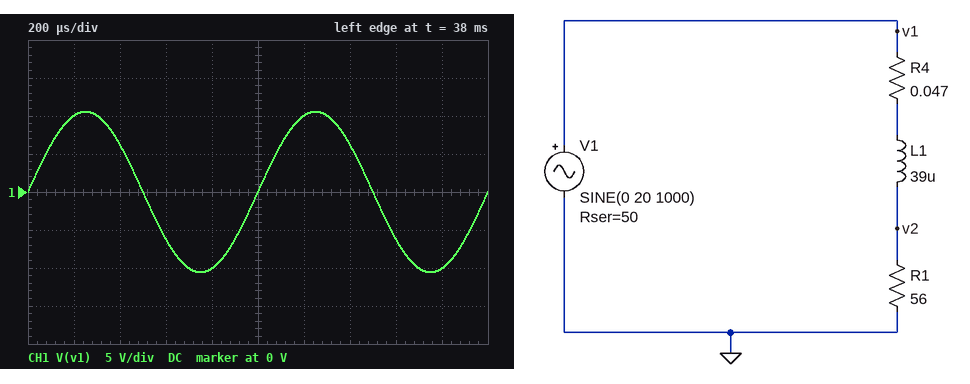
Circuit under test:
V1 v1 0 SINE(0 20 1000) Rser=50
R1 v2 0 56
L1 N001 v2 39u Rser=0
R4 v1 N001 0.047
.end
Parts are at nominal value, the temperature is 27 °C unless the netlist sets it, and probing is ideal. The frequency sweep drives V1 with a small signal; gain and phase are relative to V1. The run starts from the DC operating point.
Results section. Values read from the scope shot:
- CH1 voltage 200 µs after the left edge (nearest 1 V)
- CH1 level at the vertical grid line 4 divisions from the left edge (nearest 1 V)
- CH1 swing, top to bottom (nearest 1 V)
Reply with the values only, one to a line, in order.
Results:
10 V
-10 V
21 V
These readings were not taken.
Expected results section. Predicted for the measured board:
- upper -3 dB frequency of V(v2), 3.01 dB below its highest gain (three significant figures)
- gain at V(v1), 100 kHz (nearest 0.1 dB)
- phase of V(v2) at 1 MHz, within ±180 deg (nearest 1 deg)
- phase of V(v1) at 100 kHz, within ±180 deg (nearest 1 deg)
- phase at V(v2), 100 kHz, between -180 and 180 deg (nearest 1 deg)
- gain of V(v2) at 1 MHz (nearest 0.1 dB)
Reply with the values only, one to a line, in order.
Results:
433 kHz
-5.0 dB
-67 deg
11 deg
-13 deg
-13.6 dB
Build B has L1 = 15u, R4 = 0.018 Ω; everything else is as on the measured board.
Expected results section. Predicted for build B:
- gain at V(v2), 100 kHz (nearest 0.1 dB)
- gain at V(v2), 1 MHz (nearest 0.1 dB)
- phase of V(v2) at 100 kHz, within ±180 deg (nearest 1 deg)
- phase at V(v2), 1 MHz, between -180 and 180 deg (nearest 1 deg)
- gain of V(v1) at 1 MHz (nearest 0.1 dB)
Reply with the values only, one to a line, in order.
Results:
-5.6 dB
-8.1 dB
-5 deg
-42 deg
-2.2 dB
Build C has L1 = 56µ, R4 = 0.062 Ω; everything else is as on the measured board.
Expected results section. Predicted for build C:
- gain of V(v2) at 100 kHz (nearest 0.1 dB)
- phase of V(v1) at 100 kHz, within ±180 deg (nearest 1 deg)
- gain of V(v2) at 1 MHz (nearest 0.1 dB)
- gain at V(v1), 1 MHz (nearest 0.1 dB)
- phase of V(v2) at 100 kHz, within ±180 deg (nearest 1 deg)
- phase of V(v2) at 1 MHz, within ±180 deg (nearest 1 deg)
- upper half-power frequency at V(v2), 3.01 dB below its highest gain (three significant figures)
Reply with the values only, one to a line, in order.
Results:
-6.0 dB
14 deg
-16.3 dB
-0.3 dB
-18 deg
-73 deg
301 kHz
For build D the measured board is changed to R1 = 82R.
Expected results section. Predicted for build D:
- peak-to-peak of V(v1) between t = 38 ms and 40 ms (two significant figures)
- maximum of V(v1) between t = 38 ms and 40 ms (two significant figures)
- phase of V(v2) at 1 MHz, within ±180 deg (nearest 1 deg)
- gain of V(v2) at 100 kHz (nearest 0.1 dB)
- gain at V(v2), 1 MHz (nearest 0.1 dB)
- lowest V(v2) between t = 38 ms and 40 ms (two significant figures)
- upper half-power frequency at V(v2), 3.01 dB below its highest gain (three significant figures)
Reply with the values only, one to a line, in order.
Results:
25 V
12 V
-62 deg
-4.3 dB
-10.6 dB
-12 V
539 kHz
